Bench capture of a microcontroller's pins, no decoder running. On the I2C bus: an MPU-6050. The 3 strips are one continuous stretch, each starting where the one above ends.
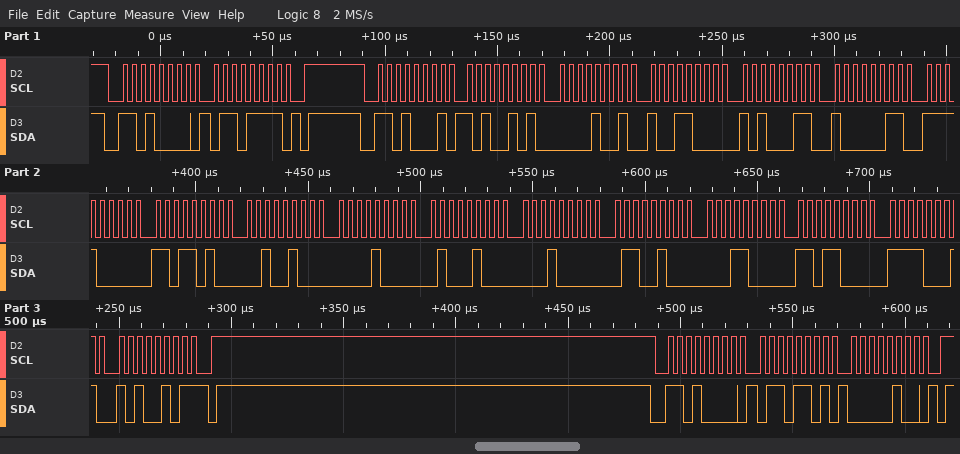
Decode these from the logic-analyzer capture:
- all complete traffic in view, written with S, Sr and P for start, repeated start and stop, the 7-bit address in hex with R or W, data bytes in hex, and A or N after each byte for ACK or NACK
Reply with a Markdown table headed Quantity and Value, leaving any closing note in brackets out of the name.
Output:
| Quantity | Value |
|---|---|
| all complete traffic in view, written with S, Sr and P for start, repeated start and stop, the 7-bit address in hex with R or W, data bytes in hex, and A or N after each byte for ACK or NACK | S 68W A 6F A P S 68R A A5 A 09 A 98 A A3 A 83 A F0 A DA A 24 A 08 A 44 A 10 A 64 A 18 A D8 A F1 A A5 N P S 68W A 6D A 04 A P |
